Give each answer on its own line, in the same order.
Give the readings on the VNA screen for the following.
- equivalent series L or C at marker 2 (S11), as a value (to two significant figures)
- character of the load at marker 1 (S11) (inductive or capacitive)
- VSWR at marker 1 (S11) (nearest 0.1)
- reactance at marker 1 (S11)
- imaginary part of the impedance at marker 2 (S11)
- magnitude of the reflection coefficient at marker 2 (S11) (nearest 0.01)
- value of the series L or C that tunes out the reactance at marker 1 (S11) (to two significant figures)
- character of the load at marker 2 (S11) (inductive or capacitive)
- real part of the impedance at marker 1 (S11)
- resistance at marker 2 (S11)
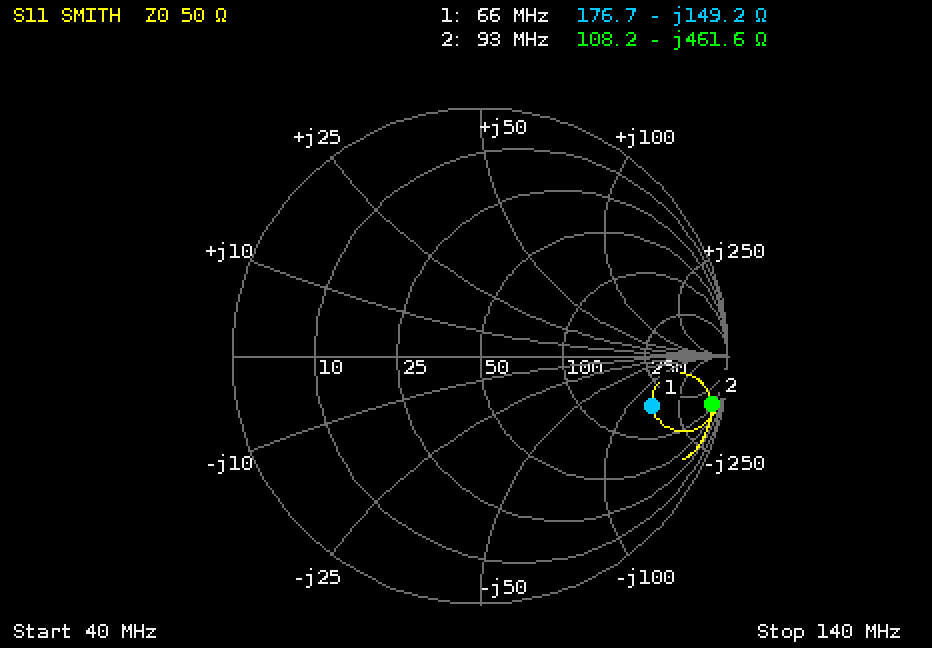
3.7 pF
capacitive
6.2
-149.2 Ω
-461.6 Ω
0.95
360 nH
capacitive
176.7 Ω
108.2 Ω
